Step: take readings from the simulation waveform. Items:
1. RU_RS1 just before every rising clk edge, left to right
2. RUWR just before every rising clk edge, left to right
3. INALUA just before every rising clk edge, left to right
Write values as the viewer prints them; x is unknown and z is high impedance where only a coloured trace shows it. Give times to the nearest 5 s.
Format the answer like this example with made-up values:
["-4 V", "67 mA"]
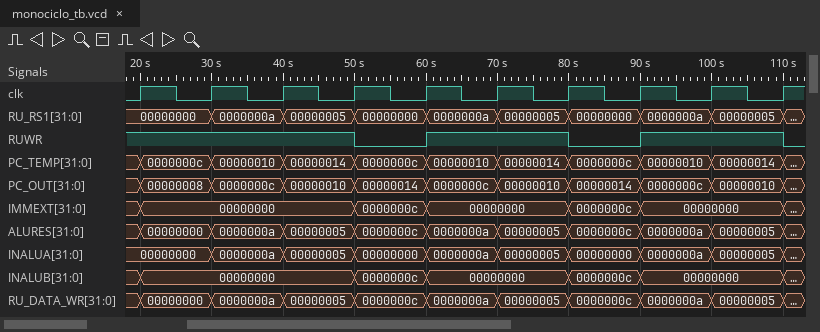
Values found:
["00000000, 00000000, 0000000a, 00000005, 00000000, 0000000a, 00000005, 00000000, 0000000a, 00000005", "1 1 1 1 0 1 1 0 1 1", "00000000, 00000000, 0000000a, 00000005, 00000000, 0000000a, 00000005, 00000000, 0000000a, 00000005"]
